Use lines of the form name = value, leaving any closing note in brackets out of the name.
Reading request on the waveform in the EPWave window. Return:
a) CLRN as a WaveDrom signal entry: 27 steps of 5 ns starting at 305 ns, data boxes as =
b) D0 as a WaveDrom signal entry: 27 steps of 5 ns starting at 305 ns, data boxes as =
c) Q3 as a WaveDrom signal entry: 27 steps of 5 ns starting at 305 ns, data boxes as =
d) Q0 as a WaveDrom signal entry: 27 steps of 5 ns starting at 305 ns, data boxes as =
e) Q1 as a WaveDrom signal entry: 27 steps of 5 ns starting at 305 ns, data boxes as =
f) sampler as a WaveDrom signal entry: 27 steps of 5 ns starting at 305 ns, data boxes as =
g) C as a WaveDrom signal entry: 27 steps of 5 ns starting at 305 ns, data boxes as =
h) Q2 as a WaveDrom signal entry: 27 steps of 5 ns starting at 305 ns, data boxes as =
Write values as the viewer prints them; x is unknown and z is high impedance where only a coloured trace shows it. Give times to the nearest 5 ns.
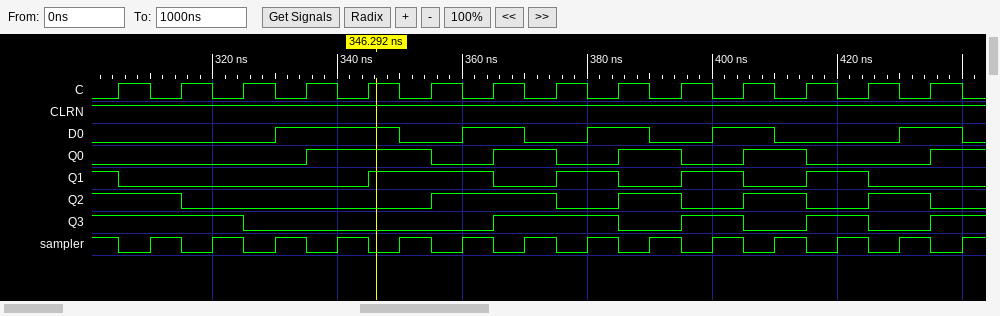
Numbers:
CLRN as a WaveDrom signal entry: 27 steps of 5 ns starting at 305 ns, data boxes as = = {name: 'CLRN', wave: '1..........................'}
D0 as a WaveDrom signal entry: 27 steps of 5 ns starting at 305 ns, data boxes as = = {name: 'D0', wave: '0....1...0.1.0.1.0.1.0...1.'}
Q3 as a WaveDrom signal entry: 27 steps of 5 ns starting at 305 ns, data boxes as = = {name: 'Q3', wave: '1...0.......1...0.1.0.1.0.1'}
Q0 as a WaveDrom signal entry: 27 steps of 5 ns starting at 305 ns, data boxes as = = {name: 'Q0', wave: '0.....1...0.1.0.1.0.1.0...1'}
Q1 as a WaveDrom signal entry: 27 steps of 5 ns starting at 305 ns, data boxes as = = {name: 'Q1', wave: '0.......1...0.1.0.1.0.1.0..'}
sampler as a WaveDrom signal entry: 27 steps of 5 ns starting at 305 ns, data boxes as = = {name: 'sampler', wave: '010101010101010101010101010'}
C as a WaveDrom signal entry: 27 steps of 5 ns starting at 305 ns, data boxes as = = {name: 'C', wave: '101010101010101010101010101'}
Q2 as a WaveDrom signal entry: 27 steps of 5 ns starting at 305 ns, data boxes as = = {name: 'Q2', wave: '1.0.......1...0.1.0.1.0.1.0'}
